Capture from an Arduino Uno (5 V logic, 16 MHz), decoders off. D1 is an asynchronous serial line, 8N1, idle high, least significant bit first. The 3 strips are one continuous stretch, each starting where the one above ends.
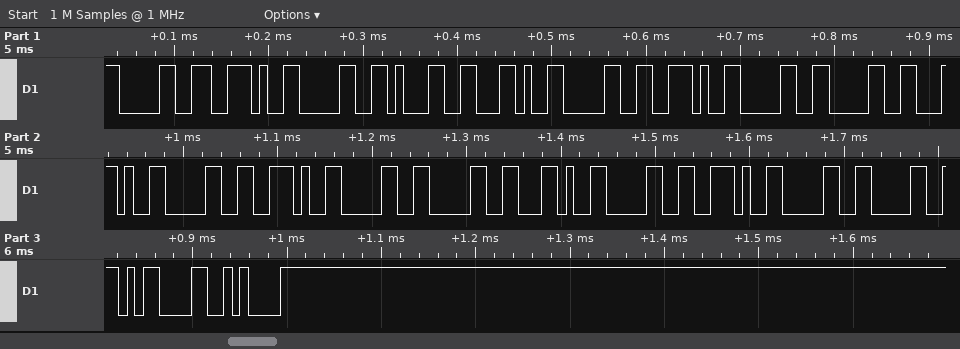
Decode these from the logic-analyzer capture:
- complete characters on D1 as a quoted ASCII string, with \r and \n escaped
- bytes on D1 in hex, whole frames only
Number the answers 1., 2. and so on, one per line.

1. "0.01,0.00,0.00,0.00\r\n"
2. 0x30 0x2E 0x30 0x31 0x2C 0x30 0x2E 0x30 0x30 0x2C 0x30 0x2E 0x30 0x30 0x2C 0x30 0x2E 0x30 0x30 0x0D 0x0A
